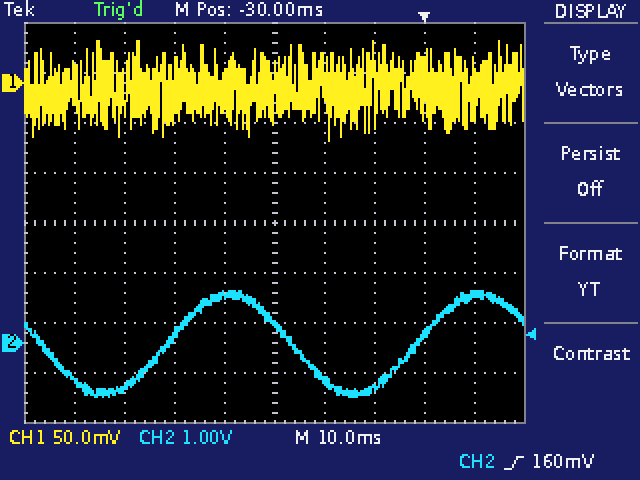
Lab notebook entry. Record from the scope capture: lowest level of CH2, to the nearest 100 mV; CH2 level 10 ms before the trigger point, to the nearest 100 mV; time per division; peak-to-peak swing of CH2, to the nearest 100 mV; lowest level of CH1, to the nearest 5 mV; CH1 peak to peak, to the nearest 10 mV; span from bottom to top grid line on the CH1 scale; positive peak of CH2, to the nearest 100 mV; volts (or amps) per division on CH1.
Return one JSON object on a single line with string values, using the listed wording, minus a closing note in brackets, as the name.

{"lowest level of CH2, to the nearest 100 mV": "-1.1 V", "CH2 level 10 ms before the trigger point, to the nearest 100 mV": "-900 mV", "time per division": "10 ms", "peak-to-peak swing of CH2, to the nearest 100 mV": "2.1 V", "lowest level of CH1, to the nearest 5 mV": "-60 mV", "CH1 peak to peak, to the nearest 10 mV": "100 mV", "span from bottom to top grid line on the CH1 scale": "400 mV", "positive peak of CH2, to the nearest 100 mV": "1.0 V", "volts (or amps) per division on CH1": "50 mV"}
